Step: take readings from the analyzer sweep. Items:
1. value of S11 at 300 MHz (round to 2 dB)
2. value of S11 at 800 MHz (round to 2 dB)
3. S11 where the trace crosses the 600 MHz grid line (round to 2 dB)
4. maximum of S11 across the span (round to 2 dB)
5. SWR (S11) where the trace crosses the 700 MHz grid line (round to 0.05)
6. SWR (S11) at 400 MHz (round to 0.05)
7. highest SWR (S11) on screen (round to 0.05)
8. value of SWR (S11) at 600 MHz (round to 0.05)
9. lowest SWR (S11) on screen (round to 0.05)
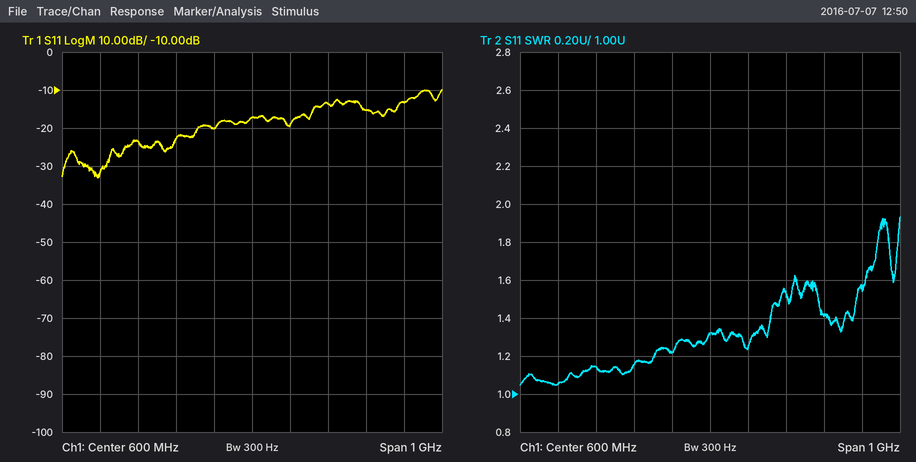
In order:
-24 dB
-14 dB
-18 dB
-10 dB
1.25
1.15
1.95
1.30
1.05
